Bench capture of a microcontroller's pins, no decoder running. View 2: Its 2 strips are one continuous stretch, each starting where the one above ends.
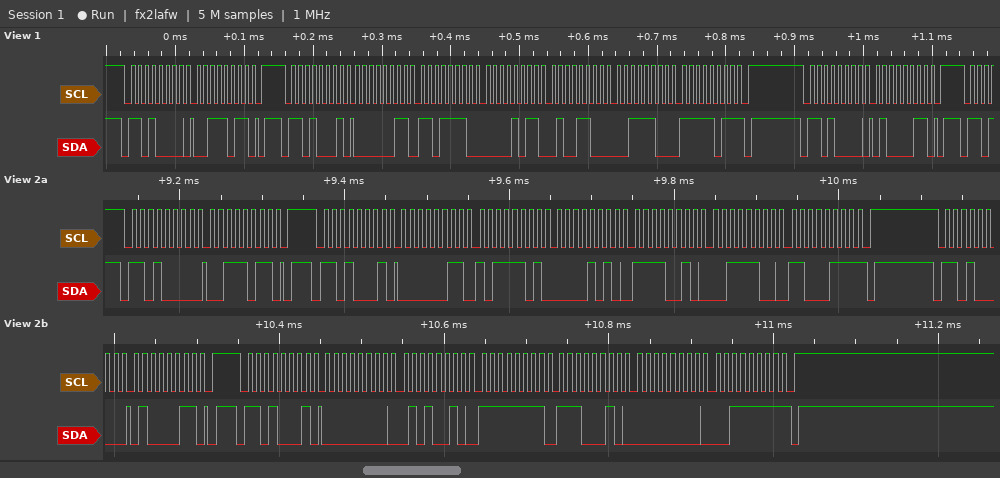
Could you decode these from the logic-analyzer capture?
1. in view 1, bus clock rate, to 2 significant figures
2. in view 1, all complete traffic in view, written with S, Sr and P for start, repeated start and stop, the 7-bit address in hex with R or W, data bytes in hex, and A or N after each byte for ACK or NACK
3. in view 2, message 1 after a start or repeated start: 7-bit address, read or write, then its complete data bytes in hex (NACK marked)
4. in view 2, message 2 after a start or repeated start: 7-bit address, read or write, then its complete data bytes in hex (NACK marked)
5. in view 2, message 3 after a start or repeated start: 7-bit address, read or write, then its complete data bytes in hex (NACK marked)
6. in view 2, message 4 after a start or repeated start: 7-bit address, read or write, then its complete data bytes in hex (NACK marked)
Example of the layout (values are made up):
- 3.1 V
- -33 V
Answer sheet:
- 100 kHz
- S 68W A 3B A P S 68R A 03 A DE A 0B A 4C A 3C A FB N P S 68W A 43 A P
- 0x68 write: 3B
- 0x68 read: 03 BD 0A F2 3C C7 NACK
- 0x68 write: 43
- 0x68 read: 00 52 FF E2 00 3F NACK
